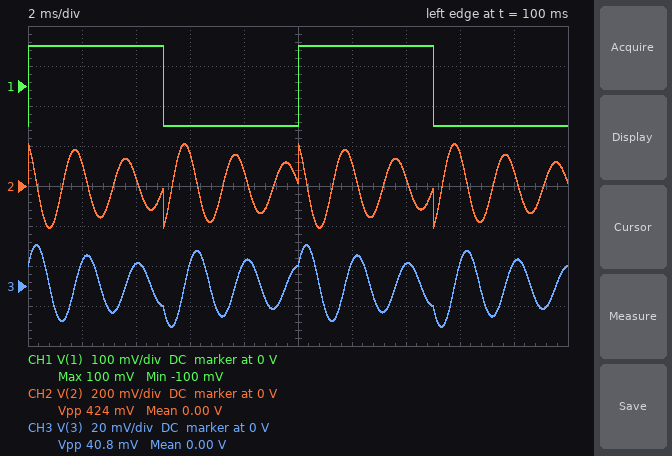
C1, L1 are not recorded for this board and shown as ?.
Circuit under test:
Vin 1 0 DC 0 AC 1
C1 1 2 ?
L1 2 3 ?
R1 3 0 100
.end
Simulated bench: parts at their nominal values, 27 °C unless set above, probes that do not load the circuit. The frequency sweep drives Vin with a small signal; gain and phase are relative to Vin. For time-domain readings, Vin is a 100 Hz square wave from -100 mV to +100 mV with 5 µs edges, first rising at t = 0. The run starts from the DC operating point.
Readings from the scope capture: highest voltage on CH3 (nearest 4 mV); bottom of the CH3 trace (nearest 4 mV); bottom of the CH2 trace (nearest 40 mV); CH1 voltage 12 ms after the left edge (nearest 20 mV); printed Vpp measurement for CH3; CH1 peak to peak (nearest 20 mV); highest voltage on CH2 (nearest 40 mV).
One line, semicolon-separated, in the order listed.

20 mV; -20 mV; -200 mV; 100 mV; 40.8 mV; 200 mV; 200 mV
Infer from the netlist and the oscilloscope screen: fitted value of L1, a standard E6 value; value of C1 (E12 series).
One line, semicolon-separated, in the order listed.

330 mH; 270 nF
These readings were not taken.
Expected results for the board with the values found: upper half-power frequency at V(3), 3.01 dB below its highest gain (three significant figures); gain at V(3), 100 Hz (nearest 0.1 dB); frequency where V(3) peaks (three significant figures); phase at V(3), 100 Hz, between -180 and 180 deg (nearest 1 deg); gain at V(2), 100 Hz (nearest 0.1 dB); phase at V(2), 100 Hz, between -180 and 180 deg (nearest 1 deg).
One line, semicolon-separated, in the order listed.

558 Hz; -35.1 dB; 533 Hz; 89 deg; -27.9 dB; 153 deg
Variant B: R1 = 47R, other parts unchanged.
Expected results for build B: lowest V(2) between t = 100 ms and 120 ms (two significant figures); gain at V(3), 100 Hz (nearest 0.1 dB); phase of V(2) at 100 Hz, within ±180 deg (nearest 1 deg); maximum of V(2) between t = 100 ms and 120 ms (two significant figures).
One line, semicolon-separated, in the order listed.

-220 mV; -41.7 dB; 167 deg; 220 mV
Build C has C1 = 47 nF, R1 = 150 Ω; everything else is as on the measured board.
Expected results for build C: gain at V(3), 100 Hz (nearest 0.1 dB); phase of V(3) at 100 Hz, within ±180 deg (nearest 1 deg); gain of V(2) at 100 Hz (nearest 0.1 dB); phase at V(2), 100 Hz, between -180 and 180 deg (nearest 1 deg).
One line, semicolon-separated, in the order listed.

-47.0 dB; 90 deg; -42.4 dB; 144 deg
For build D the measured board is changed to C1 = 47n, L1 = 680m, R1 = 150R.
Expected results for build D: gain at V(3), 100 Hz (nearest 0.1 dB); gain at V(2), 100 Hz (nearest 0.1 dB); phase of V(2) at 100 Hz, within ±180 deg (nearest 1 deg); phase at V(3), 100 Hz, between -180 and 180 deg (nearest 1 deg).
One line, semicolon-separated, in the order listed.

-47.0 dB; -37.4 dB; 160 deg; 90 deg
